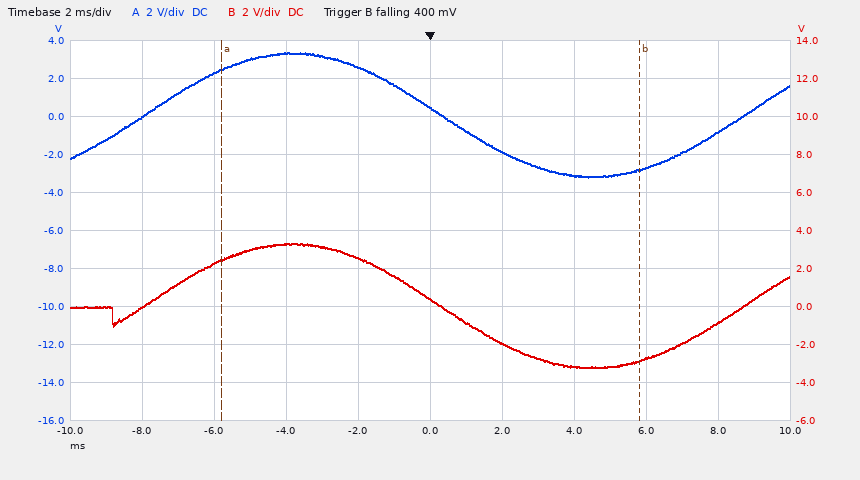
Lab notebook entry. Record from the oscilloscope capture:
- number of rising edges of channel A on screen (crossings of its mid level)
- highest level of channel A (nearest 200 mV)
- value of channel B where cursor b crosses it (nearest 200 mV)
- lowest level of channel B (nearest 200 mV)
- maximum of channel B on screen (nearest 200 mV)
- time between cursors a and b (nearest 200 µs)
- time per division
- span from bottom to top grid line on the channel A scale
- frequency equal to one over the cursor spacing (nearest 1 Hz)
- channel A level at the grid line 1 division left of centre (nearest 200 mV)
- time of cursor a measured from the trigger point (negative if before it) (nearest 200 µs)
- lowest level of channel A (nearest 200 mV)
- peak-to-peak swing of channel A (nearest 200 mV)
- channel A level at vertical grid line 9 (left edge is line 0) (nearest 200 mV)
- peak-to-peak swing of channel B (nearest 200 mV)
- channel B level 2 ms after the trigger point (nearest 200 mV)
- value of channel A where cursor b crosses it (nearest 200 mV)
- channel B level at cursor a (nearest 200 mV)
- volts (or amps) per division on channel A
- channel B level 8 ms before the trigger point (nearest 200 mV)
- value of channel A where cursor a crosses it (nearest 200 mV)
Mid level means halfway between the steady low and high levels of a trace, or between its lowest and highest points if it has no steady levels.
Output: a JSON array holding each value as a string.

["2", "3.4 V", "-2.8 V", "-3.2 V", "3.4 V", "11.6 ms", "2 ms", "20 V", "86 Hz", "2.6 V", "-5.8 ms", "-3.2 V", "6.6 V", "-800 mV", "6.6 V", "-2.0 V", "-2.8 V", "2.4 V", "2 V", "0.0 V", "2.4 V"]
